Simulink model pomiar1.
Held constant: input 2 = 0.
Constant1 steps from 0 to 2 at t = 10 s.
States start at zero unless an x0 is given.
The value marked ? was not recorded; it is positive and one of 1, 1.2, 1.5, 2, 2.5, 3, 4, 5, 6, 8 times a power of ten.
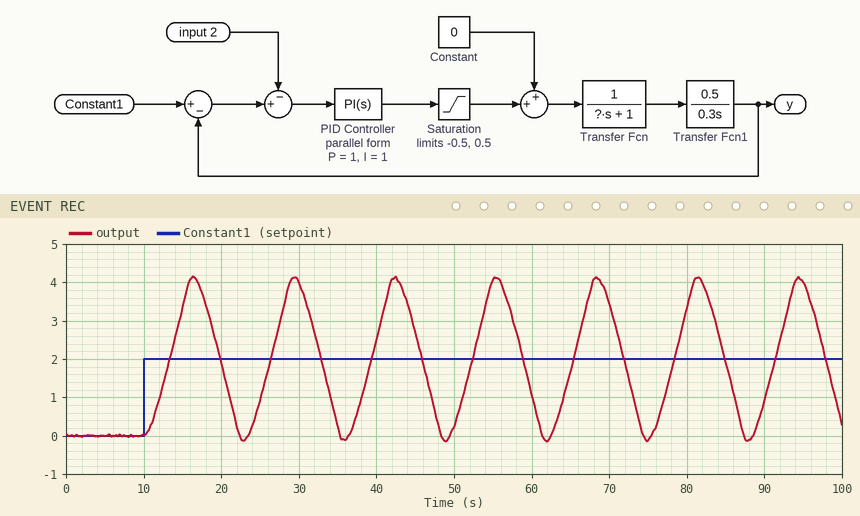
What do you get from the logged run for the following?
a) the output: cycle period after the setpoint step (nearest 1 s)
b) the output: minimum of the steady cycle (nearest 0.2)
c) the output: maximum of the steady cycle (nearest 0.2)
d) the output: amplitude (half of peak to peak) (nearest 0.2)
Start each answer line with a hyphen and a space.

- 13 s
- -0.2
- 4.2
- 2.2
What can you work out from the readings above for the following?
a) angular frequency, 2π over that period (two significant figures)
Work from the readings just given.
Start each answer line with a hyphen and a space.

- 0.48 rad/s
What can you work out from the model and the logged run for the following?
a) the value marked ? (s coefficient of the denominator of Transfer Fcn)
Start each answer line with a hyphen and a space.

- 1
